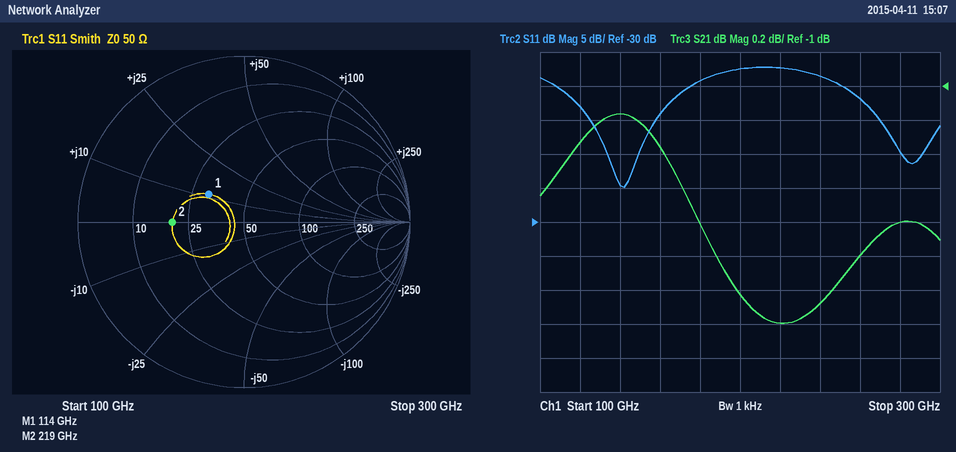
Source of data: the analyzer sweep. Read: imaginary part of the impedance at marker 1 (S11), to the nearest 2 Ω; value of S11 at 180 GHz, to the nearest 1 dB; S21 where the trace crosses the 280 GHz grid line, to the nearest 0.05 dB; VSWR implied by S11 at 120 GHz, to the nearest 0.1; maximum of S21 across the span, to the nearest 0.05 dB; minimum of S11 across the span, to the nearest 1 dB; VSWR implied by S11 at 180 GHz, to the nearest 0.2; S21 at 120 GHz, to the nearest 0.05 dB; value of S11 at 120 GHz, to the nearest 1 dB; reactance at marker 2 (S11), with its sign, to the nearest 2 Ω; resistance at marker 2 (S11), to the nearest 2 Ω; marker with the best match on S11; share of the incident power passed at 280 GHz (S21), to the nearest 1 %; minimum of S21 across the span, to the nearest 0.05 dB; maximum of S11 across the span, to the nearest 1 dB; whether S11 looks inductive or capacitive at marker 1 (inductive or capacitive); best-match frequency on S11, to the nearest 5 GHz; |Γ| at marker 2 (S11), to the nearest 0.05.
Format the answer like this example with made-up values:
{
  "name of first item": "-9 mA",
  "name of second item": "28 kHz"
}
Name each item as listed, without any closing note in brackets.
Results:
{
  "imaginary part of the impedance at marker 1 (S11), to the nearest 2 Ω": "+12 Ω",
  "value of S11 at 180 GHz, to the nearest 1 dB": "-9 dB",
  "S21 where the trace crosses the 280 GHz grid line, to the nearest 0.05 dB": "-1.80 dB",
  "VSWR implied by S11 at 120 GHz, to the nearest 0.1": "1.6",
  "maximum of S21 across the span, to the nearest 0.05 dB": "-1.15 dB",
  "minimum of S11 across the span, to the nearest 1 dB": "-25 dB",
  "VSWR implied by S11 at 180 GHz, to the nearest 0.2": "2.0",
  "S21 at 120 GHz, to the nearest 0.05 dB": "-1.35 dB",
  "value of S11 at 120 GHz, to the nearest 1 dB": "-13 dB",
  "reactance at marker 2 (S11), with its sign, to the nearest 2 Ω": "0 Ω",
  "resistance at marker 2 (S11), to the nearest 2 Ω": "20 Ω",
  "marker with the best match on S11": "marker 1",
  "share of the incident power passed at 280 GHz (S21), to the nearest 1 %": "66 %",
  "minimum of S21 across the span, to the nearest 0.05 dB": "-2.40 dB",
  "maximum of S11 across the span, to the nearest 1 dB": "-7 dB",
  "whether S11 looks inductive or capacitive at marker 1": "inductive",
  "best-match frequency on S11, to the nearest 5 GHz": "140 GHz",
  "|Γ| at marker 2 (S11), to the nearest 0.05": "0.45"
}
